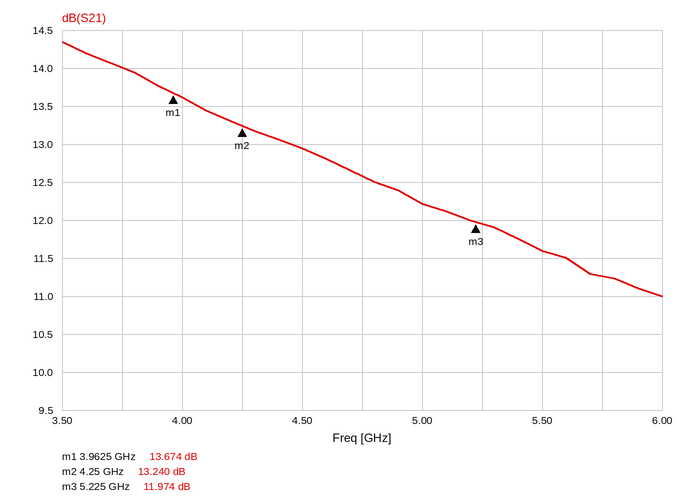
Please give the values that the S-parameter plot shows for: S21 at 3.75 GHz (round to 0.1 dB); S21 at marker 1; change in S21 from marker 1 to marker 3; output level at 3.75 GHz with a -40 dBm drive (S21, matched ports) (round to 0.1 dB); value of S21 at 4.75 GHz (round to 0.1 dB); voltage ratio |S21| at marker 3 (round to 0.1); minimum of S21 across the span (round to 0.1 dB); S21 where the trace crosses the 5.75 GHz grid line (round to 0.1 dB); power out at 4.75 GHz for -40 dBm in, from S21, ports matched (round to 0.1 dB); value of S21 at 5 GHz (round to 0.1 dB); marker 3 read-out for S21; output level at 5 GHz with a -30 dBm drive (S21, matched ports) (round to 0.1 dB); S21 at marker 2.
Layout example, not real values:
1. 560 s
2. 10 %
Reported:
1. 14.0 dB
2. 13.674 dB
3. -1.700 dB
4. -26.0 dBm
5. 12.6 dB
6. 4.0
7. 11.0 dB
8. 11.3 dB
9. -27.4 dBm
10. 12.2 dB
11. 11.974 dB
12. -17.8 dBm
13. 13.240 dB
